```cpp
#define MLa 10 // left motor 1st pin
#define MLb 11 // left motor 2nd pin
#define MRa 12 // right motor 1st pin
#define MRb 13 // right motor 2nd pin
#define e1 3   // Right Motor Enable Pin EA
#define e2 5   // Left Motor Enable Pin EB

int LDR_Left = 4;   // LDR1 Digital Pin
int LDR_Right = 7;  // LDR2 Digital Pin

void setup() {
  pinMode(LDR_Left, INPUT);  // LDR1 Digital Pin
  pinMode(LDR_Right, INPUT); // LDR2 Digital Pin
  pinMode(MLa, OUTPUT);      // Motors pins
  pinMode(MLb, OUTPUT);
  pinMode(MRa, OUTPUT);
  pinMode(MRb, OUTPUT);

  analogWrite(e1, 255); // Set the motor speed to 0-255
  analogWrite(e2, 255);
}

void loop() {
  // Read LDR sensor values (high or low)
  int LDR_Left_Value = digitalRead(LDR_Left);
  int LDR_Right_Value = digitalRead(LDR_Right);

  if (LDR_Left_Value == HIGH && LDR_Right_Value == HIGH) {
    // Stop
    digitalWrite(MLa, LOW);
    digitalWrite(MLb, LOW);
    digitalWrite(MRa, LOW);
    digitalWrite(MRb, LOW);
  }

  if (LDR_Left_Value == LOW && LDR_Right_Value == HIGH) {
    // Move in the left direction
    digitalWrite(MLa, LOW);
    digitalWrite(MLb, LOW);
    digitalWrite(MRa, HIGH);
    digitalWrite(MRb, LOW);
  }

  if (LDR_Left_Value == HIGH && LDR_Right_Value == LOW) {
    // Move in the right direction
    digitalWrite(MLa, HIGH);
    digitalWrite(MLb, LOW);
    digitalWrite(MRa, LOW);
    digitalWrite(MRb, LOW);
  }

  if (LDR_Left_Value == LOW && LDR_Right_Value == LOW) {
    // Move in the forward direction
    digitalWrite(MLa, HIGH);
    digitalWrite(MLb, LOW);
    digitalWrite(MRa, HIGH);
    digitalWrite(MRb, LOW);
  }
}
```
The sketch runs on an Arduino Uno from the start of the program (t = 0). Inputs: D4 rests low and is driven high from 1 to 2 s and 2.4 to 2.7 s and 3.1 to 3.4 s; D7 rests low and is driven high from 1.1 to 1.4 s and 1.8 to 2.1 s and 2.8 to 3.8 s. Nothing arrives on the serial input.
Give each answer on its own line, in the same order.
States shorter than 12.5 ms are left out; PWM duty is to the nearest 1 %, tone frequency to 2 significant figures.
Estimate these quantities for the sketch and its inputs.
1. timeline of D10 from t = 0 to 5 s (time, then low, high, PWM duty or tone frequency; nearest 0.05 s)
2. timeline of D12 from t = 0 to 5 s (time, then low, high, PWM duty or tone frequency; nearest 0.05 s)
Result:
0 s high; 1.1 s low; 1.4 s high; 1.8 s low; 2.1 s high; 2.8 s low; 3.8 s high
0 s high; 1 s low; 2 s high; 2.4 s low; 2.7 s high; 3.1 s low; 3.4 s high
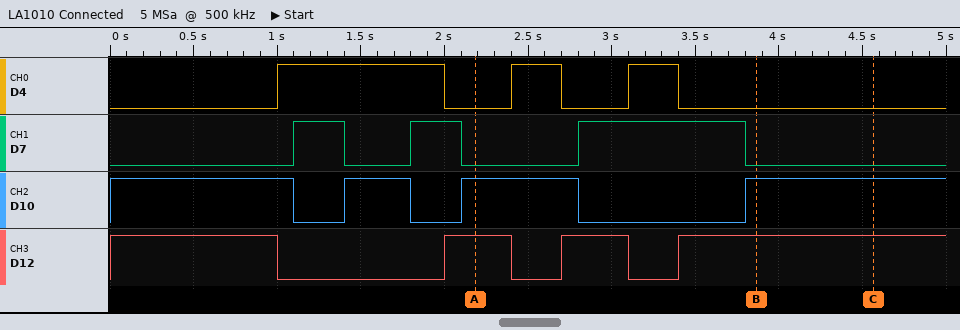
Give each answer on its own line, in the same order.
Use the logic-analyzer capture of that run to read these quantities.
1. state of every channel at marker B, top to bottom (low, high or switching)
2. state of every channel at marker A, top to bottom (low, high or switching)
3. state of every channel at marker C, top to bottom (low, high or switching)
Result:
D4 low, D7 low, D10 high, D12 high
D4 low, D7 low, D10 high, D12 high
D4 low, D7 low, D10 high, D12 high
